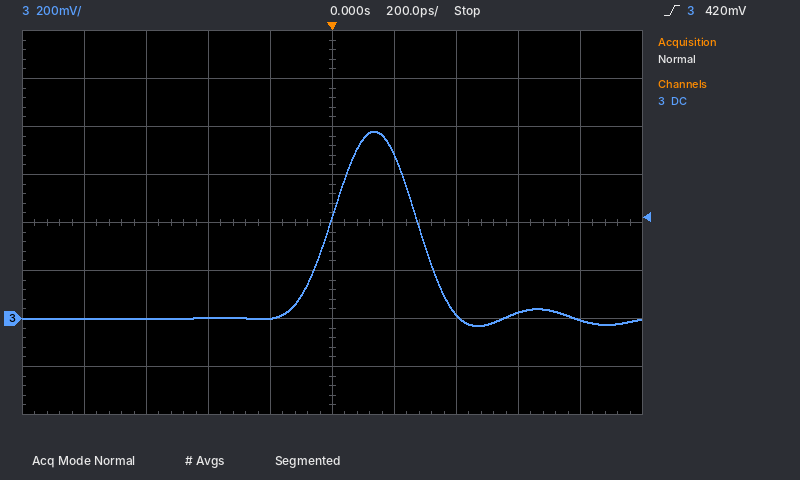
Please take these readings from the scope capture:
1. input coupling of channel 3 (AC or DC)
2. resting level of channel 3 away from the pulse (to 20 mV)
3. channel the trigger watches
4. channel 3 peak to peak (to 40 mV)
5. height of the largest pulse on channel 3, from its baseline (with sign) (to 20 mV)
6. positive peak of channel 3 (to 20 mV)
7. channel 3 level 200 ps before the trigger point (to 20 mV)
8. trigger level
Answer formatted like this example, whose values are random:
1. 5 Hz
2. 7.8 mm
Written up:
1. DC
2. 0 mV
3. channel 3
4. 800 mV
5. +780 mV
6. 780 mV
7. 0 mV
8. 420 mV
